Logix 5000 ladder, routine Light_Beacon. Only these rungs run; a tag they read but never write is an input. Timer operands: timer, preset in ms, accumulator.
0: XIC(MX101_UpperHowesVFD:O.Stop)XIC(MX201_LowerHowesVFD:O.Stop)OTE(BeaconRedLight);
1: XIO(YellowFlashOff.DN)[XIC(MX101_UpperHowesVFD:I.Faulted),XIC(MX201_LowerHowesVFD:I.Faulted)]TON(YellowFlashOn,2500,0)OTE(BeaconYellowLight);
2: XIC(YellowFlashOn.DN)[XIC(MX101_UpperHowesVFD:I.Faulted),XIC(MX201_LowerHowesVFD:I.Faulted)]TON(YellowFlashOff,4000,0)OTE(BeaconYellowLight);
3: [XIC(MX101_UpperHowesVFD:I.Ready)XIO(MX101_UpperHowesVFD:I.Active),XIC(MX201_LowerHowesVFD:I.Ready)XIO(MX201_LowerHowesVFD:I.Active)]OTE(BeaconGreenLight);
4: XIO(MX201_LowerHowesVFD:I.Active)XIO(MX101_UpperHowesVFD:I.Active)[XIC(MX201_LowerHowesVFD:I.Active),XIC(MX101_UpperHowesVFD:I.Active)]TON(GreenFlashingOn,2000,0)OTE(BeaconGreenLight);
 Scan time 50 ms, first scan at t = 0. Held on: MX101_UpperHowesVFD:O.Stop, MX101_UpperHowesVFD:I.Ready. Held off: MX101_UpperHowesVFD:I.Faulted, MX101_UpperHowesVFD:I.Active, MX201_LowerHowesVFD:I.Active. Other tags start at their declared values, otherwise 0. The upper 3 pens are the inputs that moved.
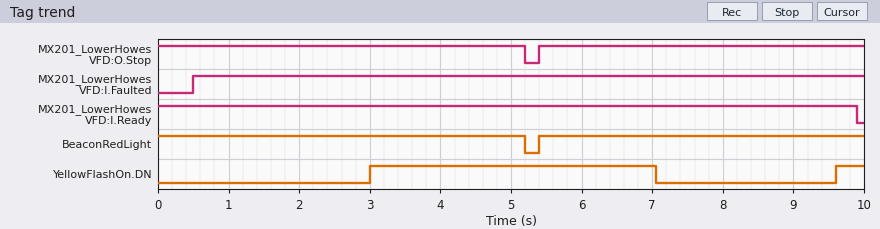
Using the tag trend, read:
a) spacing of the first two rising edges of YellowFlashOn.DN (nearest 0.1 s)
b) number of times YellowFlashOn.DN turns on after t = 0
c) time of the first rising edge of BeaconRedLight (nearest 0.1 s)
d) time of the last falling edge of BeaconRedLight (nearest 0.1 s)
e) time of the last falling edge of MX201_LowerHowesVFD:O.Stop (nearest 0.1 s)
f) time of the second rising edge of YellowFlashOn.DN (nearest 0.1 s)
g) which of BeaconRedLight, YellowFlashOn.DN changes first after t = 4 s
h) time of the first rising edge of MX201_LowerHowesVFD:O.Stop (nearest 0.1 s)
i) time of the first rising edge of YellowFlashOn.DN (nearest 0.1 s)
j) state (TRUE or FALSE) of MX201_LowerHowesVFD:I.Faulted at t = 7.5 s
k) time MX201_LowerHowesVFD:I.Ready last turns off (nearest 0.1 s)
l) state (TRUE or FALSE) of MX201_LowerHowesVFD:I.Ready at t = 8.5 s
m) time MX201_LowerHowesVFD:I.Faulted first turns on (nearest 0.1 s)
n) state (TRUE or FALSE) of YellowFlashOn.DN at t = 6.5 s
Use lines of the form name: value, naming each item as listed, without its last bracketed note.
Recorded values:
spacing of the first two rising edges of YellowFlashOn.DN: 6.6 s
number of times YellowFlashOn.DN turns on after t = 0: 2
time of the first rising edge of BeaconRedLight: 5.4 s
time of the last falling edge of BeaconRedLight: 5.2 s
time of the last falling edge of MX201_LowerHowesVFD:O.Stop: 5.2 s
time of the second rising edge of YellowFlashOn.DN: 9.6 s
which of BeaconRedLight, YellowFlashOn.DN changes first after t = 4 s: BeaconRedLight
time of the first rising edge of MX201_LowerHowesVFD:O.Stop: 5.4 s
time of the first rising edge of YellowFlashOn.DN: 3.0 s
state (TRUE or FALSE) of MX201_LowerHowesVFD:I.Faulted at t = 7.5 s: TRUE
time MX201_LowerHowesVFD:I.Ready last turns off: 9.9 s
state (TRUE or FALSE) of MX201_LowerHowesVFD:I.Ready at t = 8.5 s: TRUE
time MX201_LowerHowesVFD:I.Faulted first turns on: 0.5 s
state (TRUE or FALSE) of YellowFlashOn.DN at t = 6.5 s: TRUE
